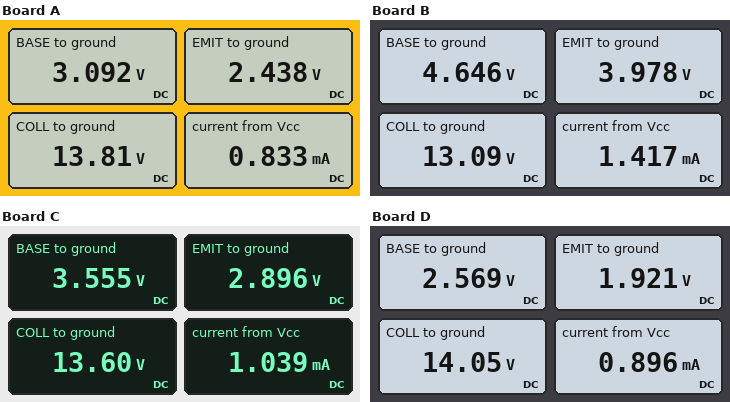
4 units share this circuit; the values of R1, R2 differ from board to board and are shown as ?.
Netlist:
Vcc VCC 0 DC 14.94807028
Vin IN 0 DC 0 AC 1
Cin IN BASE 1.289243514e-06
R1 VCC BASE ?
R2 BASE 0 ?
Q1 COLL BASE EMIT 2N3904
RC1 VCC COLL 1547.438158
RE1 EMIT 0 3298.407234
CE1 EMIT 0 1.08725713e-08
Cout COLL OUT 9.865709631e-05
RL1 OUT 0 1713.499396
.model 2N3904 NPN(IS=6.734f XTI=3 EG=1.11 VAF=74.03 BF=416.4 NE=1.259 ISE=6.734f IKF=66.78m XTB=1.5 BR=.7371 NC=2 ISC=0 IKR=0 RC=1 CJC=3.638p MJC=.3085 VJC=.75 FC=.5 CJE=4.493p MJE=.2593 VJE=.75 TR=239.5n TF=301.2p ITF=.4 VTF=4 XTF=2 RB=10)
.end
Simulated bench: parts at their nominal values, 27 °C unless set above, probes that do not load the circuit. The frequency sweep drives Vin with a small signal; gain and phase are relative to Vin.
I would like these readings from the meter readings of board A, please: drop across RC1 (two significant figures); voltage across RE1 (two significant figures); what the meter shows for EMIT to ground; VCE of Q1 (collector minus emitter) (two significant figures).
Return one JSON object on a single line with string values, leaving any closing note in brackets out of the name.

{"drop across RC1": "1.1 V", "voltage across RE1": "2.4 V", "what the meter shows for EMIT to ground": "2.438 V", "VCE of Q1 (collector minus emitter)": "11 V"}
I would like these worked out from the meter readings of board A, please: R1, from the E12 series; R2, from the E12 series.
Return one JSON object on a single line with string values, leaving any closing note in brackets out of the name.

{"R1, from the E12 series": "120 kΩ", "R2, from the E12 series": "33 kΩ"}
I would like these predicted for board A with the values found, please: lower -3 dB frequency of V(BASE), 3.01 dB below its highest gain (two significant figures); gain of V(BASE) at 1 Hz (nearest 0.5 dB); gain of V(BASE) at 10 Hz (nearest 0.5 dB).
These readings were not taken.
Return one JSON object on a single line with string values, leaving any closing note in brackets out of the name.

{"lower -3 dB frequency of V(BASE), 3.01 dB below its highest gain": "5.0 Hz", "gain of V(BASE) at 1 Hz": "-14.0 dB", "gain of V(BASE) at 10 Hz": "-1.0 dB"}
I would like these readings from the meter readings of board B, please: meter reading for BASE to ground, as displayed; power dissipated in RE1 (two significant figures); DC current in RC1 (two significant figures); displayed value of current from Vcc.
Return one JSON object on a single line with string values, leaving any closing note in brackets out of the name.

{"meter reading for BASE to ground, as displayed": "4.646 V", "power dissipated in RE1": "4.8 mW", "DC current in RC1": "1.2 mA", "displayed value of current from Vcc": "1.417 mA"}
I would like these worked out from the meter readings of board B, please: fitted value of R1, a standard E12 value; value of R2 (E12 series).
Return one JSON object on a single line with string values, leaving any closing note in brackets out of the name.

{"fitted value of R1, a standard E12 value": "47 kΩ", "value of R2": "22 kΩ"}
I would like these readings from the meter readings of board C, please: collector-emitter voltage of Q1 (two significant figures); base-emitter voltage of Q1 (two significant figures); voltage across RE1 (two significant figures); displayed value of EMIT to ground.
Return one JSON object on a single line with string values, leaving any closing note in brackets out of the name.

{"collector-emitter voltage of Q1": "11 V", "base-emitter voltage of Q1": "660 mV", "voltage across RE1": "2.9 V", "displayed value of EMIT to ground": "2.896 V"}
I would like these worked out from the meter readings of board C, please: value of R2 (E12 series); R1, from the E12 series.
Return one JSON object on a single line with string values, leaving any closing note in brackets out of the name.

{"value of R2": "22 kΩ", "R1, from the E12 series": "68 kΩ"}
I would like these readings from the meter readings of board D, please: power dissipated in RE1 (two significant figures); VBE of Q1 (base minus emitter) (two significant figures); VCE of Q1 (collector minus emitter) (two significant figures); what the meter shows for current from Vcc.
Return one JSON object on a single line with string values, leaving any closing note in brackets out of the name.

{"power dissipated in RE1": "1.1 mW", "VBE of Q1 (base minus emitter)": "650 mV", "VCE of Q1 (collector minus emitter)": "12 V", "what the meter shows for current from Vcc": "0.896 mA"}
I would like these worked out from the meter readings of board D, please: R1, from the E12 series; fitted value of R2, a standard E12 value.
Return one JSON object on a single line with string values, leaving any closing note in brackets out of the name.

{"R1, from the E12 series": "39 kΩ", "fitted value of R2, a standard E12 value": "8.2 kΩ"}
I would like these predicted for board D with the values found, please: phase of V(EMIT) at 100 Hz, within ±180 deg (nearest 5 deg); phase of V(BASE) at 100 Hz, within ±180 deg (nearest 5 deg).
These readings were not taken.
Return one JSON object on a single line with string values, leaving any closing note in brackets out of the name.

{"phase of V(EMIT) at 100 Hz, within ±180 deg": "10 deg", "phase of V(BASE) at 100 Hz, within ±180 deg": "10 deg"}
